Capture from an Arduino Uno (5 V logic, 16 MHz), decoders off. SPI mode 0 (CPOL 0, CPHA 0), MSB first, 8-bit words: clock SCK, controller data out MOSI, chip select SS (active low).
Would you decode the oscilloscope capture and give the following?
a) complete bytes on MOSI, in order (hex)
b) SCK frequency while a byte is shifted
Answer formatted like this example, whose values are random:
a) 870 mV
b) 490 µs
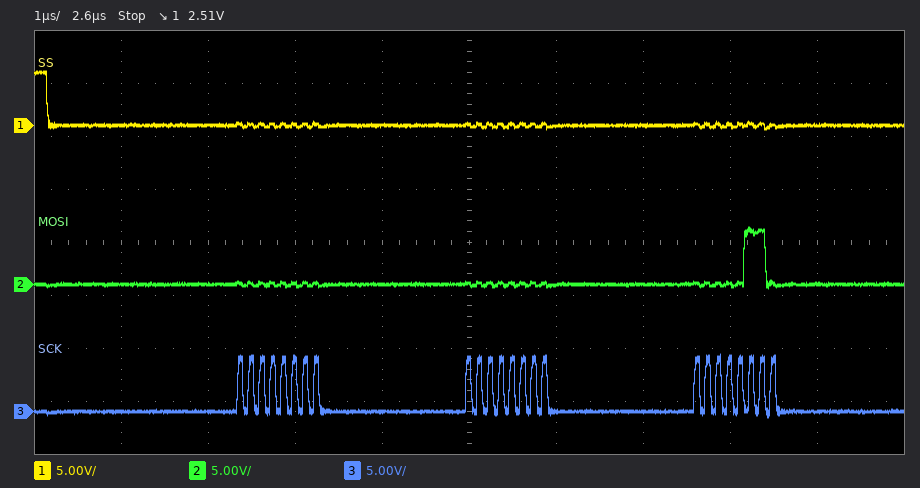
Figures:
a) 0x00 0x00 0x06
b) 8 MHz
